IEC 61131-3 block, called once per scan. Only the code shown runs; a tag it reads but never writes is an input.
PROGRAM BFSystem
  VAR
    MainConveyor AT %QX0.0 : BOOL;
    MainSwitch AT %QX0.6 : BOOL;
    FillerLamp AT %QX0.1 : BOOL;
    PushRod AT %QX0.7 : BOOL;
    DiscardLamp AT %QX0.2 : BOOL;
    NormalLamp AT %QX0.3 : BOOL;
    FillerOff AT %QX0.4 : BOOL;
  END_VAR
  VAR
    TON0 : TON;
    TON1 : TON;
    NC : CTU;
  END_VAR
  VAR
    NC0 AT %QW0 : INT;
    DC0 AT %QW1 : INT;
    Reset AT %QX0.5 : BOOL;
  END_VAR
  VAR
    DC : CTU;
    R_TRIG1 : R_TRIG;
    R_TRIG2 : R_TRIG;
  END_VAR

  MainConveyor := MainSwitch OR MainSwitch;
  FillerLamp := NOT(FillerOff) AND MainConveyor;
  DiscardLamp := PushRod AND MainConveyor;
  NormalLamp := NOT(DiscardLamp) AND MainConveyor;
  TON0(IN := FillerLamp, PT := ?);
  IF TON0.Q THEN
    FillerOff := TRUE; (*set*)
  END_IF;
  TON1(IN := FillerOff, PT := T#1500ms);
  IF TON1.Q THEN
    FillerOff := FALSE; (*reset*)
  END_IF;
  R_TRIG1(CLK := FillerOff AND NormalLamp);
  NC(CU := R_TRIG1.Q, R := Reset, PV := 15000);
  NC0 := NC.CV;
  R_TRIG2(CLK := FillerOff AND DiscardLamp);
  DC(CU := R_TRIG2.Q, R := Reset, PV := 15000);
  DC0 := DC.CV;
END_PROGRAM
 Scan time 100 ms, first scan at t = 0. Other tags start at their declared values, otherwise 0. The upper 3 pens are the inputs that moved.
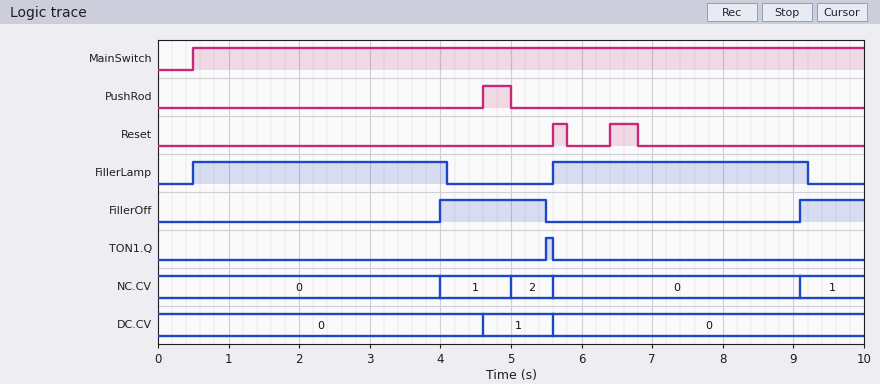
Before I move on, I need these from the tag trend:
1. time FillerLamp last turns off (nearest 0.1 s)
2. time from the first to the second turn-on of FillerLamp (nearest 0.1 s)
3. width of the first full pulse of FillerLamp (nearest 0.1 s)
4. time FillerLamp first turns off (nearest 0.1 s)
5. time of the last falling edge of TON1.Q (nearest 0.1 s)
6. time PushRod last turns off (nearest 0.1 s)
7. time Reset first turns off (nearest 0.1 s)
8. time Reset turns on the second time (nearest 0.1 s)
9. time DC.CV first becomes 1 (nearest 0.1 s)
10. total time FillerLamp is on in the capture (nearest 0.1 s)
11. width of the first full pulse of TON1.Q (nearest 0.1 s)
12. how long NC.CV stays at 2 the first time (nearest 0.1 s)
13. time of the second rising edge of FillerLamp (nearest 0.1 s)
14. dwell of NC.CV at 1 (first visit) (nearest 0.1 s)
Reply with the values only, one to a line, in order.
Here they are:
9.2 s
5.1 s
3.6 s
4.1 s
5.6 s
5.0 s
5.8 s
6.4 s
4.6 s
7.2 s
0.1 s
0.6 s
5.6 s
1.0 s
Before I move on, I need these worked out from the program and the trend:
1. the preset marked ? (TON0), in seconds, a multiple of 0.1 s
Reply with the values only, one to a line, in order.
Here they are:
3.5 s
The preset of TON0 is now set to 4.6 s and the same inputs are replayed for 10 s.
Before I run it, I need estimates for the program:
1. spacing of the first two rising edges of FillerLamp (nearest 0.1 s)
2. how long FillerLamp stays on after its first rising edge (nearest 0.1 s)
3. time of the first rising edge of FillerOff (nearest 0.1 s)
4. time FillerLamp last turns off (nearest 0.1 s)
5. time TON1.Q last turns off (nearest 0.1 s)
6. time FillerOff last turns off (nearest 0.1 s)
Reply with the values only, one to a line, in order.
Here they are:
6.2 s
4.7 s
5.1 s
5.2 s
6.7 s
6.6 s
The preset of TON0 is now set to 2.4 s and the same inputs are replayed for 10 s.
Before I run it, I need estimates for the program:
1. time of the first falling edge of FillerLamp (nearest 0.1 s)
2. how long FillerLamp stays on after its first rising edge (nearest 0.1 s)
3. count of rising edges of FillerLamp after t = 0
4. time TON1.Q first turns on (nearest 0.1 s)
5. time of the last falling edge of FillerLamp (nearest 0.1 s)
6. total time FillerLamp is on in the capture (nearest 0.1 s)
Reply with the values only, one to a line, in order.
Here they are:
3.0 s
2.5 s
3
4.4 s
7.0 s
6.5 s
